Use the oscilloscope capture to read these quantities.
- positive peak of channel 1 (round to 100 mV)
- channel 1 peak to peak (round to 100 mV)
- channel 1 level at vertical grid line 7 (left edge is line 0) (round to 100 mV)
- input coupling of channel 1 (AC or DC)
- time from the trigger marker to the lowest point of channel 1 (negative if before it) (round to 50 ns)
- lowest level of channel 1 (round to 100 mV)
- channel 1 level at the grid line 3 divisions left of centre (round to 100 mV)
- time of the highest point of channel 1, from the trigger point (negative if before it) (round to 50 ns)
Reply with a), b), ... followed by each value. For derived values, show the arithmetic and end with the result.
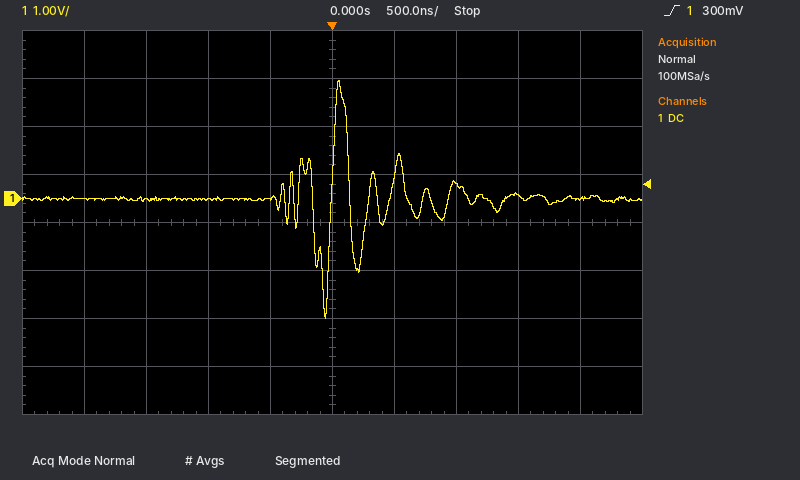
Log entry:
a) 2.5 V
b) 2.5 V − (-2.5 V) = 5.0 V
c) 300 mV
d) DC
e) -50 ns
f) -2.5 V
g) 0.0 V
h) +50 ns
